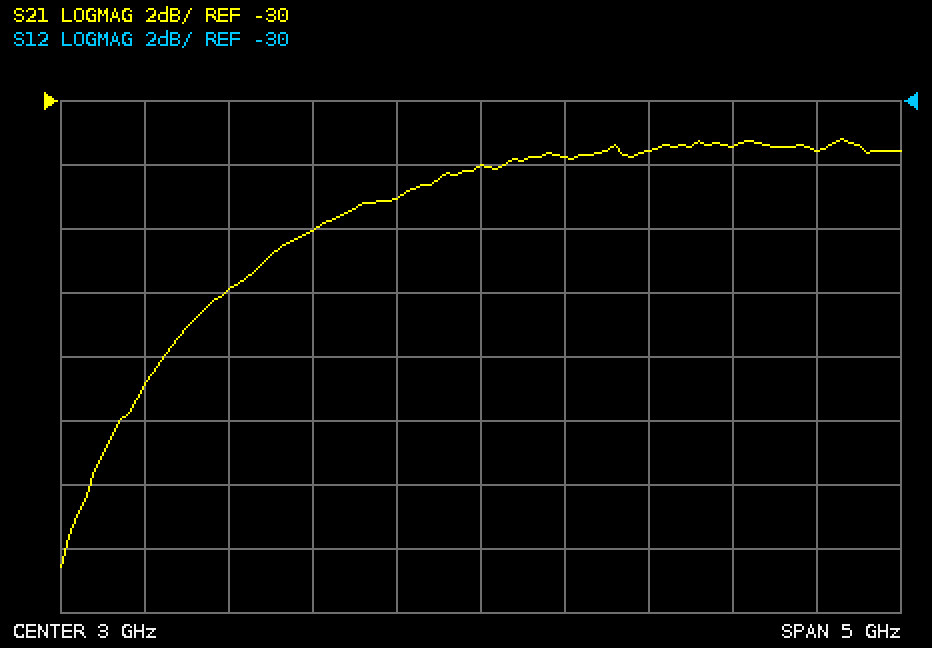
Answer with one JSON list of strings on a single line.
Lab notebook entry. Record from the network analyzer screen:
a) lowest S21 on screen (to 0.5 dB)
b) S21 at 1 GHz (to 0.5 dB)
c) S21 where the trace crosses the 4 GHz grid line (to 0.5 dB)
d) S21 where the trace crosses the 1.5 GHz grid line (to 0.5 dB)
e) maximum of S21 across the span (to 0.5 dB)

["-44.5 dB", "-39.0 dB", "-31.5 dB", "-36.0 dB", "-31.0 dB"]
